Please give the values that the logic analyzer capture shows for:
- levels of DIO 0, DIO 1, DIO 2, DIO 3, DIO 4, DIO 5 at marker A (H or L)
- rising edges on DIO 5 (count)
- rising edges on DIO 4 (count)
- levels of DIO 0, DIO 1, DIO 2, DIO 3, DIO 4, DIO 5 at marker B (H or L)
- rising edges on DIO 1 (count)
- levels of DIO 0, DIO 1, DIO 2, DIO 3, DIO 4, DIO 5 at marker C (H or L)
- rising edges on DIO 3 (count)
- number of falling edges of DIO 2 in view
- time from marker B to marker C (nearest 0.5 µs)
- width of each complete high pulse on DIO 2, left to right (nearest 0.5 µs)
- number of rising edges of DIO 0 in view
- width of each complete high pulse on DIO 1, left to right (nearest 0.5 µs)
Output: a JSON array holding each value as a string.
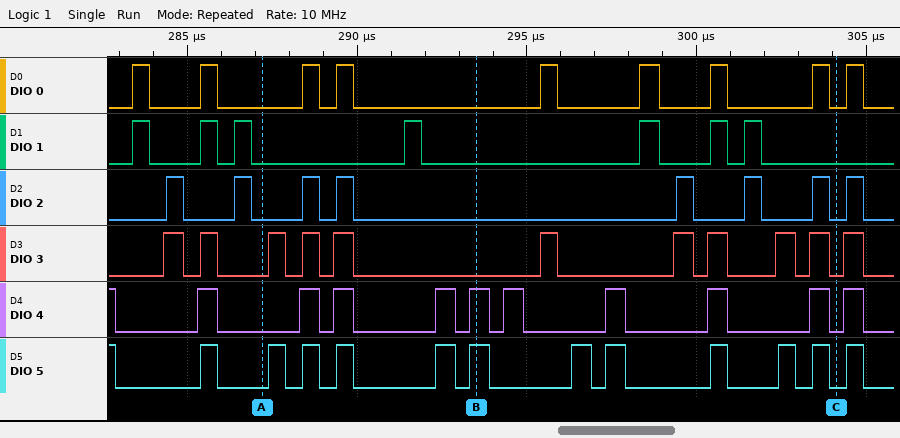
["DIO 0=L, DIO 1=L, DIO 2=L, DIO 3=L, DIO 4=L, DIO 5=L", "12", "10", "DIO 0=L, DIO 1=L, DIO 2=L, DIO 3=L, DIO 4=H, DIO 5=H", "7", "DIO 0=L, DIO 1=L, DIO 2=L, DIO 3=L, DIO 4=L, DIO 5=L", "11", "8", "10.5 µs", "0.5 µs, 0.5 µs, 0.5 µs, 0.5 µs, 0.5 µs, 0.5 µs, 0.5 µs, 0.5 µs", "9", "0.5 µs, 0.5 µs, 0.5 µs, 0.5 µs, 0.5 µs, 0.5 µs, 0.5 µs"]
